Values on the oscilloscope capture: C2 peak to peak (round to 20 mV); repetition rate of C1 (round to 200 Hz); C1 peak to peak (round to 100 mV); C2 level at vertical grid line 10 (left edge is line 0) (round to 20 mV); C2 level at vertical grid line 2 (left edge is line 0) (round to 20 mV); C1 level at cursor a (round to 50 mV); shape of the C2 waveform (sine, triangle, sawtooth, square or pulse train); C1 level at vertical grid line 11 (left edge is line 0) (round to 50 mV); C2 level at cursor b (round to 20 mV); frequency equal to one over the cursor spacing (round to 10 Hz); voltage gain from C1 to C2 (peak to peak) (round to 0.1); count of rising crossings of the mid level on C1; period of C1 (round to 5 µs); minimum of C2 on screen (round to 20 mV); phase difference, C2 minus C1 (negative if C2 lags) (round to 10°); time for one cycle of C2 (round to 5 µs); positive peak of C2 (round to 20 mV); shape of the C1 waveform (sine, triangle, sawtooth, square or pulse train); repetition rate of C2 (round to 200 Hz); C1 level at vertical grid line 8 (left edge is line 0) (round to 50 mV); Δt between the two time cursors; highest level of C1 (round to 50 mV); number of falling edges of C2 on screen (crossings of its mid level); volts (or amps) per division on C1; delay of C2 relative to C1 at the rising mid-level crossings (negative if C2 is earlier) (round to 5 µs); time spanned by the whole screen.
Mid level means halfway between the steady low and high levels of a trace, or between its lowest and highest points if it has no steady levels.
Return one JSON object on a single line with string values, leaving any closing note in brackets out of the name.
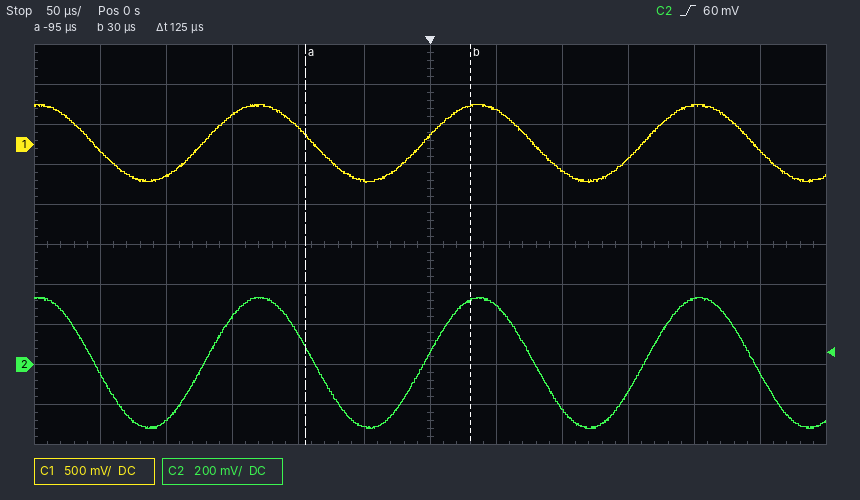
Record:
{"C2 peak to peak": "660 mV", "repetition rate of C1": "6.0 kHz", "C1 peak to peak": "1.00 V", "C2 level at vertical grid line 10 (left edge is line 0)": "320 mV", "C2 level at vertical grid line 2 (left edge is line 0)": "-280 mV", "C1 level at cursor a": "100 mV", "shape of the C2 waveform": "sine", "C1 level at vertical grid line 11 (left edge is line 0)": "-100 mV", "C2 level at cursor b": "320 mV", "frequency equal to one over the cursor spacing": "8.00 kHz", "voltage gain from C1 to C2 (peak to peak)": "0.7", "count of rising crossings of the mid level on C1": "3", "period of C1": "165 µs", "minimum of C2 on screen": "-320 mV", "phase difference, C2 minus C1 (negative if C2 lags)": "0°", "time for one cycle of C2": "165 µs", "positive peak of C2": "340 mV", "shape of the C1 waveform": "sine", "repetition rate of C2": "6.0 kHz", "C1 level at vertical grid line 8 (left edge is line 0)": "-350 mV", "Δt between the two time cursors": "125 µs", "highest level of C1": "500 mV", "number of falling edges of C2 on screen": "4", "volts (or amps) per division on C1": "500 mV", "delay of C2 relative to C1 at the rising mid-level crossings (negative if C2 is earlier)": "0 µs", "time spanned by the whole screen": "600 µs"}
